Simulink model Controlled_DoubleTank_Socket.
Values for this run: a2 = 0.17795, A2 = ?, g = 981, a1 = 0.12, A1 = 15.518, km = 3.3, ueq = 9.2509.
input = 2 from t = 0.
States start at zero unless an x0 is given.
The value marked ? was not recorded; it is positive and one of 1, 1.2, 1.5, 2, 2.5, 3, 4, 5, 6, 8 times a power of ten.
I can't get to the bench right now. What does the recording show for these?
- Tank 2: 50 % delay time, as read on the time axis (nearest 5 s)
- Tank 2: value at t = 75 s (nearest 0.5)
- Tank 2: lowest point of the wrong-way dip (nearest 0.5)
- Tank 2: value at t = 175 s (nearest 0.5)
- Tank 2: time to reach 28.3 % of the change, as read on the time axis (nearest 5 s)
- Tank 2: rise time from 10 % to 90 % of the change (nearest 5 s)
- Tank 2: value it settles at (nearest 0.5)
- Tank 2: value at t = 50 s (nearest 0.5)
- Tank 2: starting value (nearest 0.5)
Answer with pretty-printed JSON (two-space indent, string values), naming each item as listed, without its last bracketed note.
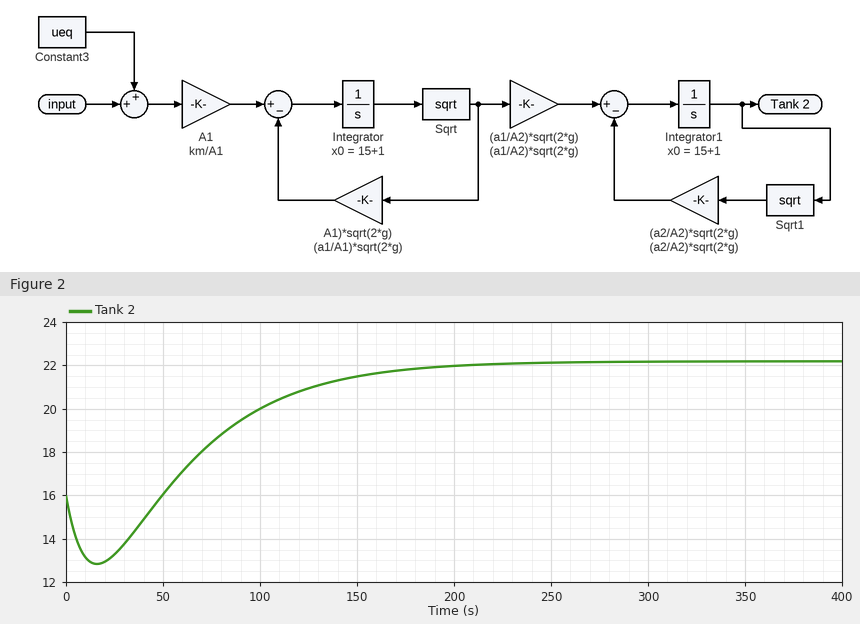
{
  "Tank 2: 50 % delay time, as read on the time axis": "85 s",
  "Tank 2: value at t = 75 s": "18.5",
  "Tank 2: lowest point of the wrong-way dip": "13.0",
  "Tank 2: value at t = 175 s": "22.0",
  "Tank 2: time to reach 28.3 % of the change, as read on the time axis": "65 s",
  "Tank 2: rise time from 10 % to 90 % of the change": "100 s",
  "Tank 2: value it settles at": "22.0",
  "Tank 2: value at t = 50 s": "16.0",
  "Tank 2: starting value": "16.0"
}
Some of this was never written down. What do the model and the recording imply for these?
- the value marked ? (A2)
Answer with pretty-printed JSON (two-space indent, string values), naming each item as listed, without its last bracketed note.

{
  "the value marked ?": "20"
}
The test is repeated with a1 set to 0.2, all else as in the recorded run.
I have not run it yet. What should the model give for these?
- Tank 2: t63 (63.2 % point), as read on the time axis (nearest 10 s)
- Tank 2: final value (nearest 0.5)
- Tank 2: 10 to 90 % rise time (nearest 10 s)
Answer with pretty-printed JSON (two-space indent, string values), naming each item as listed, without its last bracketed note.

{
  "Tank 2: t63 (63.2 % point), as read on the time axis": "30 s",
  "Tank 2: final value": "22.0",
  "Tank 2: 10 to 90 % rise time": "60 s"
}
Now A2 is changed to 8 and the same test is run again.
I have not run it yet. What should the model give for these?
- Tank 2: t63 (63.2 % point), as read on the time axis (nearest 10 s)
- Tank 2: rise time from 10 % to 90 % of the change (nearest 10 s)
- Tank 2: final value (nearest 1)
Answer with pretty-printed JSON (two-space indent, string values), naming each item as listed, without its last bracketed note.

{
  "Tank 2: t63 (63.2 % point), as read on the time axis": "80 s",
  "Tank 2: rise time from 10 % to 90 % of the change": "90 s",
  "Tank 2: final value": "22"
}
